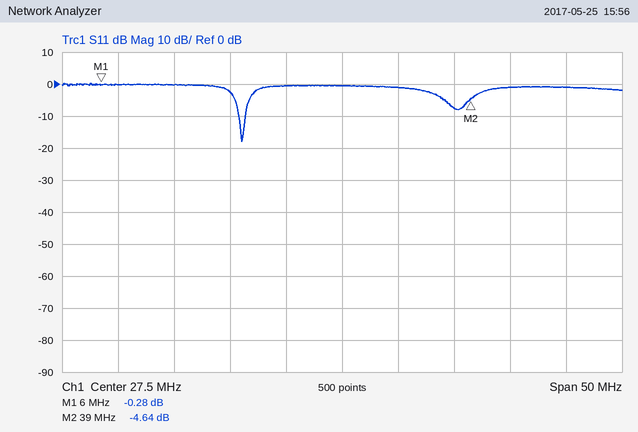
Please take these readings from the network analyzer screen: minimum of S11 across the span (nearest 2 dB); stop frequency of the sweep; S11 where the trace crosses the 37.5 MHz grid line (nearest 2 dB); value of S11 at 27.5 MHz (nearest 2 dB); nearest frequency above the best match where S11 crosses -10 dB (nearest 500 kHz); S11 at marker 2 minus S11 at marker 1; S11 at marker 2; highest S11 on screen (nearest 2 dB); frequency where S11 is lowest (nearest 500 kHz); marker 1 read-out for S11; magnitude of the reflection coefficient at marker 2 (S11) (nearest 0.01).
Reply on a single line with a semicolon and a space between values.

-18 dB; 52.5 MHz; -8 dB; 0 dB; 19.0 MHz; -4.36 dB; -4.64 dB; 0 dB; 18.5 MHz; -0.28 dB; 0.59
